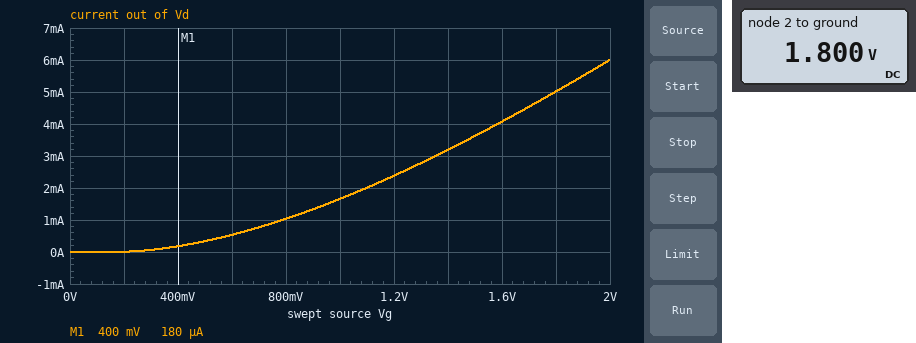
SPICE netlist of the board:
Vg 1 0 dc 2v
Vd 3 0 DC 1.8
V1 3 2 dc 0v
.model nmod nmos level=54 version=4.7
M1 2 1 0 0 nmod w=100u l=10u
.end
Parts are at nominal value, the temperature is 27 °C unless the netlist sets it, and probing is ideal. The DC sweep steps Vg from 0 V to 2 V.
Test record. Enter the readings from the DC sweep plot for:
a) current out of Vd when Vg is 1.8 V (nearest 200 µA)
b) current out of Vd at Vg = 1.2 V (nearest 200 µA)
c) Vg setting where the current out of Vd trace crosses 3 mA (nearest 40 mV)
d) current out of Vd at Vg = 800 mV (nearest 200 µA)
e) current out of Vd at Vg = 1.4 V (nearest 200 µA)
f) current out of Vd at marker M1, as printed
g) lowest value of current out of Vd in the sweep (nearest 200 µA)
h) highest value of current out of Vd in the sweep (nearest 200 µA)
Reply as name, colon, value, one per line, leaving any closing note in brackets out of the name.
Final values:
current out of Vd when Vg is 1.8 V: 5.0 mA
current out of Vd at Vg = 1.2 V: 2.4 mA
Vg setting where the current out of Vd trace crosses 3 mA: 1.36 V
current out of Vd at Vg = 800 mV: 1.0 mA
current out of Vd at Vg = 1.4 V: 3.2 mA
current out of Vd at marker M1, as printed: 180 µA
lowest value of current out of Vd in the sweep: 0 A
highest value of current out of Vd in the sweep: 6.0 mA
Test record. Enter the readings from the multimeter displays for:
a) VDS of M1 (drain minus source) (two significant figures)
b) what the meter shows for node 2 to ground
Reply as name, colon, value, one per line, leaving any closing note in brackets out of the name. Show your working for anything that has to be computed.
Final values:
VDS of M1 (drain minus source): 1.8 V = 1.8 V
what the meter shows for node 2 to ground: 1.800 V
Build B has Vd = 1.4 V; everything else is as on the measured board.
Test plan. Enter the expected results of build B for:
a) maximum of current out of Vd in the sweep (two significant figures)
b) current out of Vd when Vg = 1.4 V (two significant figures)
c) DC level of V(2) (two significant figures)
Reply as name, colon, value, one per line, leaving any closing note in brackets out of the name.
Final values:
maximum of current out of Vd in the sweep: 5.8 mA
current out of Vd when Vg = 1.4 V: 3.2 mA
DC level of V(2): 1.4 V
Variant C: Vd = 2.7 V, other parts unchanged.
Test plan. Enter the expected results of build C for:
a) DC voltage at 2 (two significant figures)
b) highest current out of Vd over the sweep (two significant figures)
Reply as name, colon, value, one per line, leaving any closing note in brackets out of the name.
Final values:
DC voltage at 2: 2.7 V
highest current out of Vd over the sweep: 6.1 mA
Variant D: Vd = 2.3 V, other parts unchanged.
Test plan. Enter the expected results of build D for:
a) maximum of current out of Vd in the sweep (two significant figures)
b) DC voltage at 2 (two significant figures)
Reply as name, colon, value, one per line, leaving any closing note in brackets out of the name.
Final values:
maximum of current out of Vd in the sweep: 6.1 mA
DC voltage at 2: 2.3 V
